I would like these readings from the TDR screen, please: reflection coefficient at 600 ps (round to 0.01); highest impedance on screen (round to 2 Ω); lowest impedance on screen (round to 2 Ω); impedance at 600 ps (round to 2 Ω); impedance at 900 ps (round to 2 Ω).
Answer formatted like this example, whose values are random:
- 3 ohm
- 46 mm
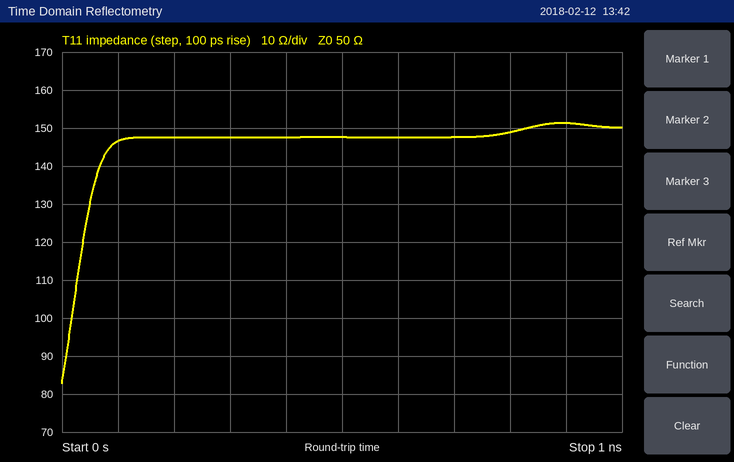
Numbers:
- +0.49
- 152 Ω
- 82 Ω
- 148 Ω
- 152 Ω
